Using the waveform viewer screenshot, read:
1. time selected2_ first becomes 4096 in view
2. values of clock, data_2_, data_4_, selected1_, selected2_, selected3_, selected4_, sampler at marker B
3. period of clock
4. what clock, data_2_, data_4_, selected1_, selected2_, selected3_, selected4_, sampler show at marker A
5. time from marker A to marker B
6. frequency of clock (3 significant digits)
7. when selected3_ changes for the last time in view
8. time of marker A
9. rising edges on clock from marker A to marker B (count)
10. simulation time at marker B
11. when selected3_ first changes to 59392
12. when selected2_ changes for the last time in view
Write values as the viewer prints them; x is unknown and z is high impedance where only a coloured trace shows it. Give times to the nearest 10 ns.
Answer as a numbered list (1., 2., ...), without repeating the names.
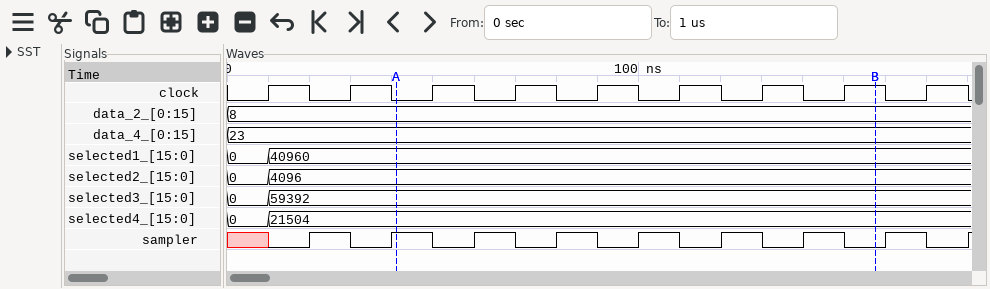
1. 10 ns
2. clock=1, data_2_=8, data_4_=23, selected1_=40960, selected2_=4096, selected3_=59392, selected4_=21504, sampler=0
3. 20 ns
4. clock=0, data_2_=8, data_4_=23, selected1_=40960, selected2_=4096, selected3_=59392, selected4_=21504, sampler=1
5. 120 ns
6. 50.0 MHz
7. 10 ns
8. 40 ns
9. 6
10. 160 ns
11. 10 ns
12. 10 ns
